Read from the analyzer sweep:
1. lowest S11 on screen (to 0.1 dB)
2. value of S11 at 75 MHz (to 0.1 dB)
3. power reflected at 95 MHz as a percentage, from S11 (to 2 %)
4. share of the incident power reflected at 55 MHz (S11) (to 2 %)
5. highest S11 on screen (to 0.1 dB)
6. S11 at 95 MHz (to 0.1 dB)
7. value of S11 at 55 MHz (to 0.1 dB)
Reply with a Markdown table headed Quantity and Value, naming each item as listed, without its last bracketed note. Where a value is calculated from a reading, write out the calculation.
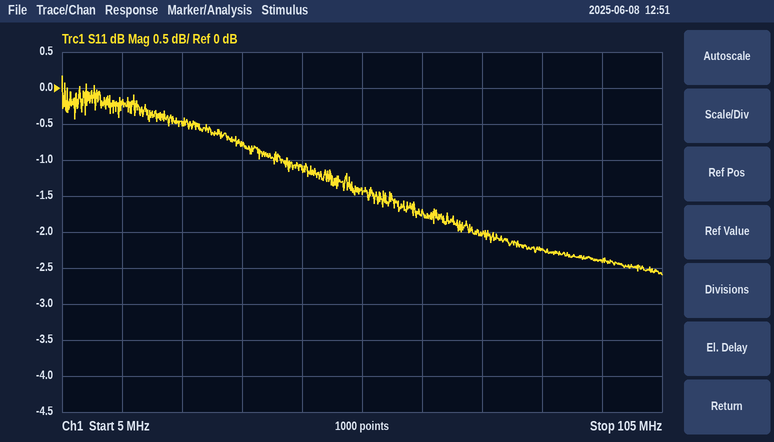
| Quantity | Value |
|---|---|
| lowest S11 on screen | -2.6 dB |
| value of S11 at 75 MHz | -2.0 dB |
| power reflected at 95 MHz as a percentage, from S11 | 10^(-2.4/10) ≈ 58 % |
| share of the incident power reflected at 55 MHz (S11) | 10^(-1.4/10) ≈ 72 % |
| highest S11 on screen | 0.2 dB |
| S11 at 95 MHz | -2.4 dB |
| value of S11 at 55 MHz | -1.4 dB |
